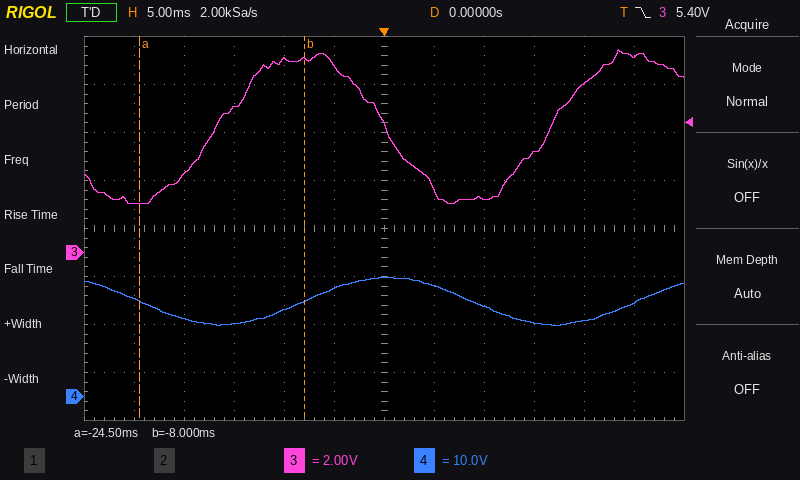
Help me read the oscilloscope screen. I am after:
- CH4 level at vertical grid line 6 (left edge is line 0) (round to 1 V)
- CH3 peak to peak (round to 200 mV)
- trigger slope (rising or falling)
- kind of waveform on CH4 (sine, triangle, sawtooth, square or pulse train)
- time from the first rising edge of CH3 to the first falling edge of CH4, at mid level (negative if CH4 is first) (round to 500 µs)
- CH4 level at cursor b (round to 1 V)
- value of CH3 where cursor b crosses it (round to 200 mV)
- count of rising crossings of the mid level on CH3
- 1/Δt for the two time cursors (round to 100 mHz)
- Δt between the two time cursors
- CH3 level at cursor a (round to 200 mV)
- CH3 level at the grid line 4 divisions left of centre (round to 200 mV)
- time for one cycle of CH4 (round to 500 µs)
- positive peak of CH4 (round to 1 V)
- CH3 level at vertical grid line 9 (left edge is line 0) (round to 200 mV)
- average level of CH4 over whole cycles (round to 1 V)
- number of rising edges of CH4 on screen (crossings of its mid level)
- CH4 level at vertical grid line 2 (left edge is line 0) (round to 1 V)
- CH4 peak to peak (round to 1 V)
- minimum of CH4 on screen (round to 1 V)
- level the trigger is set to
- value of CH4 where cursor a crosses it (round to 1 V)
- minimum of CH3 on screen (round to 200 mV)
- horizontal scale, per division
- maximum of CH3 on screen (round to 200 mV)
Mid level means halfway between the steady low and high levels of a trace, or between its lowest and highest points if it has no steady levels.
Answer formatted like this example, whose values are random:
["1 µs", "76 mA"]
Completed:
["25 V", "6.4 V", "falling", "sine", "-7.5 ms", "20 V", "8.0 V", "2", "60.6 Hz", "16.5 ms", "2.0 V", "3.2 V", "33.0 ms", "25 V", "4.2 V", "20 V", "2", "16 V", "10 V", "15 V", "5.40 V", "20 V", "2.0 V", "5 ms", "8.4 V"]
